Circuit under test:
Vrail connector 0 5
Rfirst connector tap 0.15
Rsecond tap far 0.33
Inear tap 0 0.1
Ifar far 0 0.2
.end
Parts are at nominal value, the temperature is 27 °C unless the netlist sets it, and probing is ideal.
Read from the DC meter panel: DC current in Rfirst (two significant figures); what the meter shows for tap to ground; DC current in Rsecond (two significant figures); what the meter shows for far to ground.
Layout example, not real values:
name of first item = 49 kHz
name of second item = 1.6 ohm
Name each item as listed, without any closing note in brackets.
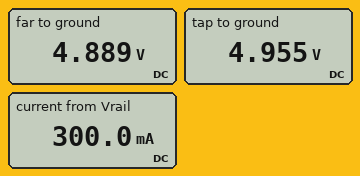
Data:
DC current in Rfirst = 300 mA
what the meter shows for tap to ground = 4.955 V
DC current in Rsecond = 200 mA
what the meter shows for far to ground = 4.889 V
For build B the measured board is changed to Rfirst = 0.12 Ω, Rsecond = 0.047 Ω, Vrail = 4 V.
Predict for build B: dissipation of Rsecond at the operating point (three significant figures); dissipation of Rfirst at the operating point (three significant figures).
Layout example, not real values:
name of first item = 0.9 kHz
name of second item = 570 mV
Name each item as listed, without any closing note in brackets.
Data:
dissipation of Rsecond at the operating point = 1.88 mW
dissipation of Rfirst at the operating point = 10.8 mW
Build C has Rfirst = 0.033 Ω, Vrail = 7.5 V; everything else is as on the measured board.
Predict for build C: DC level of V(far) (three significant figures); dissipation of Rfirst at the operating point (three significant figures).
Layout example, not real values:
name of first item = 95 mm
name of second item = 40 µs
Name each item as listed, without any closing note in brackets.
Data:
DC level of V(far) = 7.42 V
dissipation of Rfirst at the operating point = 2.97 mW
